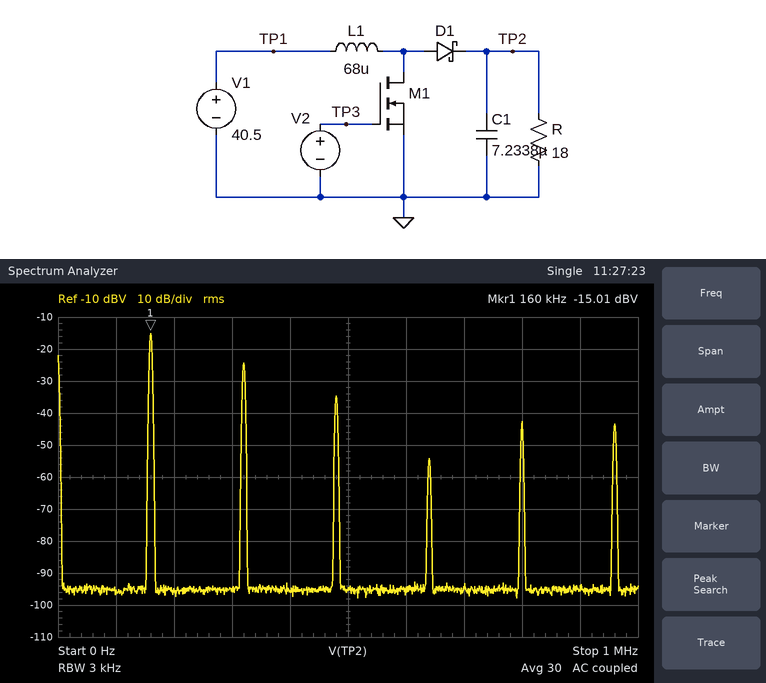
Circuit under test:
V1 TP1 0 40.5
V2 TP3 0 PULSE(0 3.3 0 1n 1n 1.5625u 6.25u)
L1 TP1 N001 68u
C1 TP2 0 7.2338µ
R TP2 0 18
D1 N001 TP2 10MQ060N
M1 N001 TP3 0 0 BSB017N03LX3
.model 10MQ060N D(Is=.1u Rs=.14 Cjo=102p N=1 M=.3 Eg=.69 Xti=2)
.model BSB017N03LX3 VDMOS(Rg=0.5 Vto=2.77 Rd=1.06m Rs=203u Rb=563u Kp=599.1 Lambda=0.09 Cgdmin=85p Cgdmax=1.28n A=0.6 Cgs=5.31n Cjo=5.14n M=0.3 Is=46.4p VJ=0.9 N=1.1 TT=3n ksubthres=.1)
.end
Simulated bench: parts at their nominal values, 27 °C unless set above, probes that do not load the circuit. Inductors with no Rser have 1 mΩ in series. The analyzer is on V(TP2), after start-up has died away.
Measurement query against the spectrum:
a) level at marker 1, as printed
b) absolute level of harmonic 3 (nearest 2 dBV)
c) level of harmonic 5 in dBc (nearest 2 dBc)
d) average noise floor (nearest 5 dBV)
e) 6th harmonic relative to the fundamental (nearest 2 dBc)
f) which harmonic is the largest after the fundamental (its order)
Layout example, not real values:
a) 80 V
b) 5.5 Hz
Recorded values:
a) -15.01 dBV
b) -34 dBV
c) -28 dBc
d) -95 dBV
e) -28 dBc
f) 2
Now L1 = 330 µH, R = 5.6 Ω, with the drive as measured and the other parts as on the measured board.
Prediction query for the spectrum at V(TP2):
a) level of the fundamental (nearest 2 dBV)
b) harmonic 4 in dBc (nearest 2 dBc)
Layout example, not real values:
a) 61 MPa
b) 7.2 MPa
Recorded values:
a) -6 dBV
b) -58 dBc
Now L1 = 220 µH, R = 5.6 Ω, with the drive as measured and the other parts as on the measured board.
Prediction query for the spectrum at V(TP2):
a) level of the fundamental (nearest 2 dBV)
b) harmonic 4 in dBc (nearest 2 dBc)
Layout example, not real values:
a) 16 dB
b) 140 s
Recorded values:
a) -6 dBV
b) -56 dBc
